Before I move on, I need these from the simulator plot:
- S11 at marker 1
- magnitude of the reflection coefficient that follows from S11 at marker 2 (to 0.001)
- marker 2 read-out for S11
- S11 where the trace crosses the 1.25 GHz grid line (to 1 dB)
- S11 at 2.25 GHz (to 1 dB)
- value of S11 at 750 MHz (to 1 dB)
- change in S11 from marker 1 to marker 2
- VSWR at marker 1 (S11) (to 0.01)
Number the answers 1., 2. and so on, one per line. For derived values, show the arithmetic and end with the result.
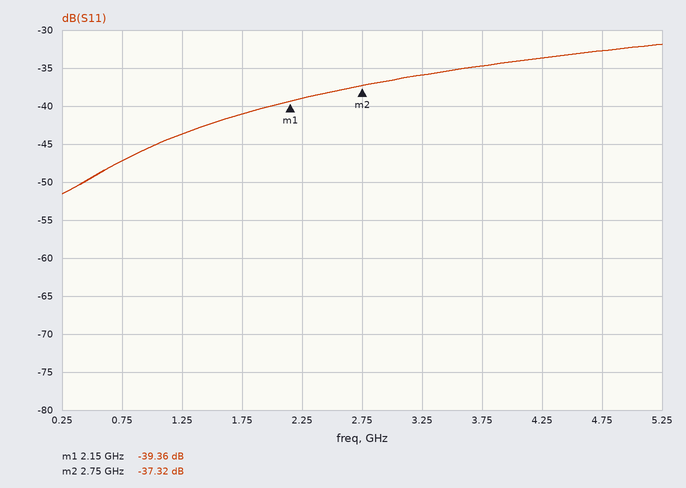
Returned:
1. -39.36 dB
2. 10^(-37.32/20) ≈ 0.014
3. -37.32 dB
4. -44 dB
5. -39 dB
6. -47 dB
7. -37.32 − (-39.36) = 2.04 dB
8. (1 + 0.0108)/(1 − 0.0108) ≈ 1.02
